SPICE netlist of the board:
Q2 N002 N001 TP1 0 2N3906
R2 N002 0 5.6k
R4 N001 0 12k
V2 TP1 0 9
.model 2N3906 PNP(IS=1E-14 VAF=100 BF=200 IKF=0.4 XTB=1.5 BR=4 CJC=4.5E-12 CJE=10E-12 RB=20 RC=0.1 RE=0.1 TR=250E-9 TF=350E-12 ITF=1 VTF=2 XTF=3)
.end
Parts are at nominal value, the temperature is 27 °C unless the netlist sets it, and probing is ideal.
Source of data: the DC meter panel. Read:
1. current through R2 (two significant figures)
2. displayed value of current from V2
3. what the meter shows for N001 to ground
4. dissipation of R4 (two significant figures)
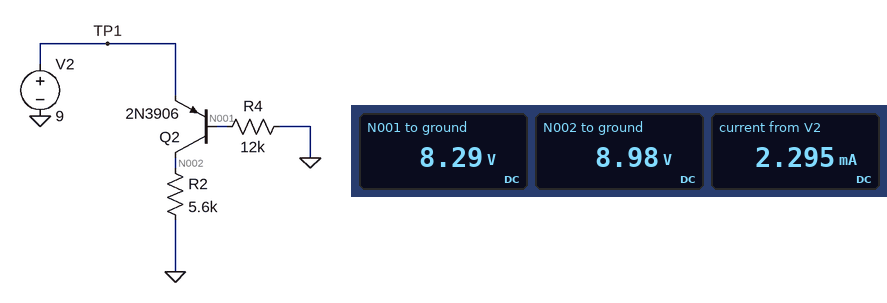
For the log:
1.6 mA
2.295 mA
8.29 V
5.7 mW
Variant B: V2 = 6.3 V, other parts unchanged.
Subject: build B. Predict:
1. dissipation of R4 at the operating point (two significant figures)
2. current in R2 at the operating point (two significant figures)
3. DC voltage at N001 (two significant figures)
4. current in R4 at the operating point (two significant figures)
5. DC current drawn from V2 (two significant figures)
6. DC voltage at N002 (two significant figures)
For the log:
2.6 mW
1.1 mA
5.6 V
470 µA
1.6 mA
6.3 V
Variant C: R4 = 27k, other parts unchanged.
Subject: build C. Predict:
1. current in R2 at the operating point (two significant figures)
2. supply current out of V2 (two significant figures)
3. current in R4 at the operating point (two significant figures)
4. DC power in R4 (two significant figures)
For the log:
1.6 mA
1.9 mA
310 µA
2.6 mW
